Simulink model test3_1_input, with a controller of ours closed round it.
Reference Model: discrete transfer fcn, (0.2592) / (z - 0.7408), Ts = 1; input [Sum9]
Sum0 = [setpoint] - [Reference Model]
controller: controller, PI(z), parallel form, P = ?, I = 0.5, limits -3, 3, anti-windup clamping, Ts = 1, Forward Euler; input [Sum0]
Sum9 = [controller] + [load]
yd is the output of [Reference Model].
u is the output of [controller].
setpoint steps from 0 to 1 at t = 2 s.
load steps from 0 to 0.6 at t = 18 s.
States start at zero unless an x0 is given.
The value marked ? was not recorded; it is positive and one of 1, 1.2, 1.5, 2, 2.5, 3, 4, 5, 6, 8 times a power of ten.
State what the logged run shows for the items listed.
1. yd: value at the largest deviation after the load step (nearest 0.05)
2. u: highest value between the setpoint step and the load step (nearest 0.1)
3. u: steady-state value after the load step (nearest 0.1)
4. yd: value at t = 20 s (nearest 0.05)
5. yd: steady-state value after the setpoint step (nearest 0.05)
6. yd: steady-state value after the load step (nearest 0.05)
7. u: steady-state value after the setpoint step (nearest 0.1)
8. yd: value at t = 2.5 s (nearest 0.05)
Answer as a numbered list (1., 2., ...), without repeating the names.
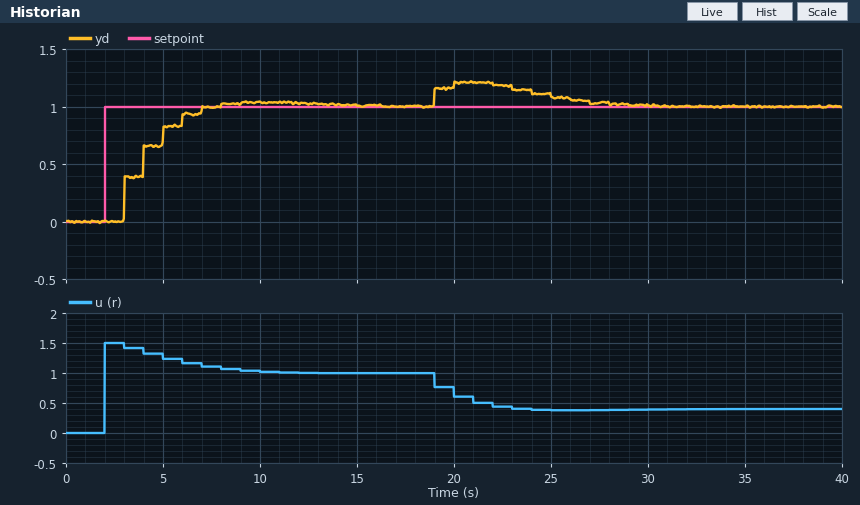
1. 1.20
2. 1.5
3. 0.4
4. 1.20
5. 1.00
6. 1.00
7. 1.0
8. 0.00
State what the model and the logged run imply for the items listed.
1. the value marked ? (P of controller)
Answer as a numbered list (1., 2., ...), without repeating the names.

1. 1.5
